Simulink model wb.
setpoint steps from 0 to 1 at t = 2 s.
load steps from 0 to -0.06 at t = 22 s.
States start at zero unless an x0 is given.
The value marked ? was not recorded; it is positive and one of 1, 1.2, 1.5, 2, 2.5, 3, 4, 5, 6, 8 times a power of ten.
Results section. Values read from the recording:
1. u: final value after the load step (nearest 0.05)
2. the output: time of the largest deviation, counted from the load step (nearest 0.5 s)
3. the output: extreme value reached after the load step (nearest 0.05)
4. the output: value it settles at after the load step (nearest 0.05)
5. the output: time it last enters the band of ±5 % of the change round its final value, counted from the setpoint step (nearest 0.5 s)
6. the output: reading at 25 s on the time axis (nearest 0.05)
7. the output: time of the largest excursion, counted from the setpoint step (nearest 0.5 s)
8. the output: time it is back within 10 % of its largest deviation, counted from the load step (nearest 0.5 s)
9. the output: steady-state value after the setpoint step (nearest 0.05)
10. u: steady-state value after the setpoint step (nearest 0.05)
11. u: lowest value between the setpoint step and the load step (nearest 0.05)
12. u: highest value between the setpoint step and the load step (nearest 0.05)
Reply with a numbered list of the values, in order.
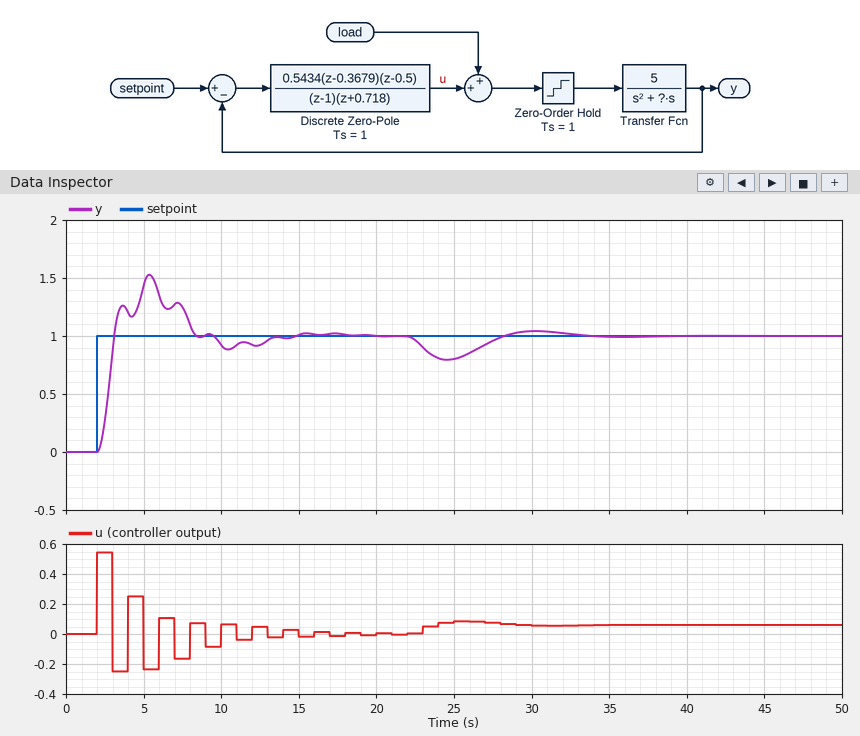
1. 0.05
2. 2.5 s
3. 0.80
4. 1.00
5. 11.0 s
6. 0.80
7. 3.5 s
8. 10.5 s
9. 1.00
10. 0.00
11. -0.25
12. 0.55
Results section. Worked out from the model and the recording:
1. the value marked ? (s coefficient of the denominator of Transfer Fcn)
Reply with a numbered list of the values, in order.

1. 1.5
